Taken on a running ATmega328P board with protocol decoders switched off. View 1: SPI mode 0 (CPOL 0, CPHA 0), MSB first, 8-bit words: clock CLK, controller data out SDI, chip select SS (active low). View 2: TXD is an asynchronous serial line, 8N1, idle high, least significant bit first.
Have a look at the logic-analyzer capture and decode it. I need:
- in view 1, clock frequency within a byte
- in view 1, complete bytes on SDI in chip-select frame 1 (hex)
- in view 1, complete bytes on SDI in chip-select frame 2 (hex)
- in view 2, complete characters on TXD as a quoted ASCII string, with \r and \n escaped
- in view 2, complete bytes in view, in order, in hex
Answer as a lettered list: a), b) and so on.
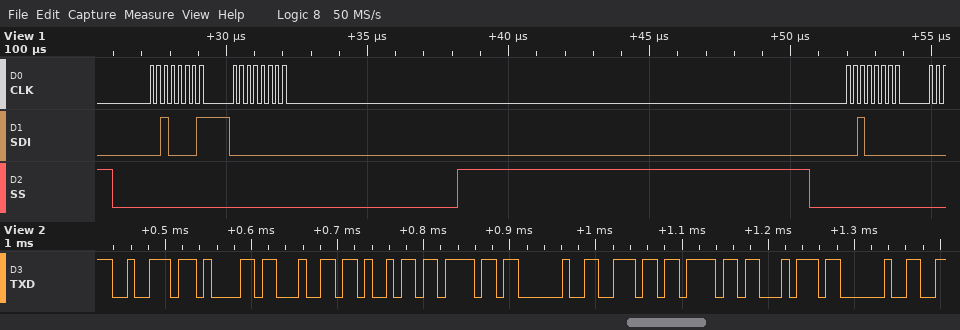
a) 4 MHz
b) 21 00
c) 20
d) "radio not "
e) 72 61 64 69 6F 20 6E 6F 74 20
